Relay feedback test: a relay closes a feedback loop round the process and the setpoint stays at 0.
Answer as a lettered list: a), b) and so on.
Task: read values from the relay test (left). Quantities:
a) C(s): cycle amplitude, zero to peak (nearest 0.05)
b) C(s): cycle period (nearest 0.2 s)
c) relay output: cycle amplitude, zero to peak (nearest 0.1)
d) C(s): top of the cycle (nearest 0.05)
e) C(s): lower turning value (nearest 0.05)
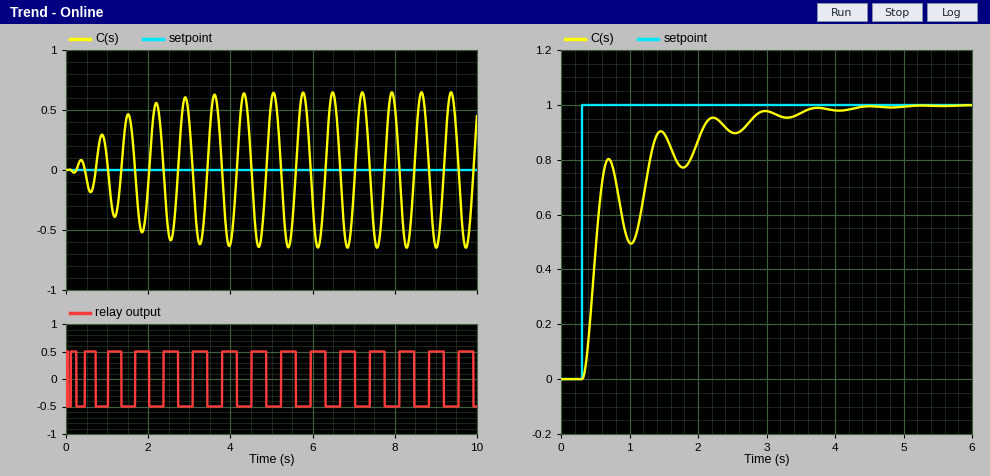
a) 0.65
b) 0.8 s
c) 0.5
d) 0.65
e) -0.65
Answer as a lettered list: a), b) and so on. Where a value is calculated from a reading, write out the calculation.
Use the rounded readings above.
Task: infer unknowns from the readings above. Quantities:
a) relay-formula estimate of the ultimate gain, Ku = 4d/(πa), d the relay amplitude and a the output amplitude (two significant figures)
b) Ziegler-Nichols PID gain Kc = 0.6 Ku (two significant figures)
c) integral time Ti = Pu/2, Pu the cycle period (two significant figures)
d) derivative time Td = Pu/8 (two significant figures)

a) 4 × 0.5 / (π × 0.65) = 0.98
b) 0.6 × 0.98 = 0.59
c) 0.8 / 2 = 0.40 s
d) 0.8 / 8 = 0.10 s
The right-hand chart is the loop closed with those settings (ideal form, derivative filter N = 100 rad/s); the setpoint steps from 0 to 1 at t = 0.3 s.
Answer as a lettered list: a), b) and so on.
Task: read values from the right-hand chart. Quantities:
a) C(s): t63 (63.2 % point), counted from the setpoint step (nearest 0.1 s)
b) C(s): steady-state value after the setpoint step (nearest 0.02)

a) 0.3 s
b) 1.00
